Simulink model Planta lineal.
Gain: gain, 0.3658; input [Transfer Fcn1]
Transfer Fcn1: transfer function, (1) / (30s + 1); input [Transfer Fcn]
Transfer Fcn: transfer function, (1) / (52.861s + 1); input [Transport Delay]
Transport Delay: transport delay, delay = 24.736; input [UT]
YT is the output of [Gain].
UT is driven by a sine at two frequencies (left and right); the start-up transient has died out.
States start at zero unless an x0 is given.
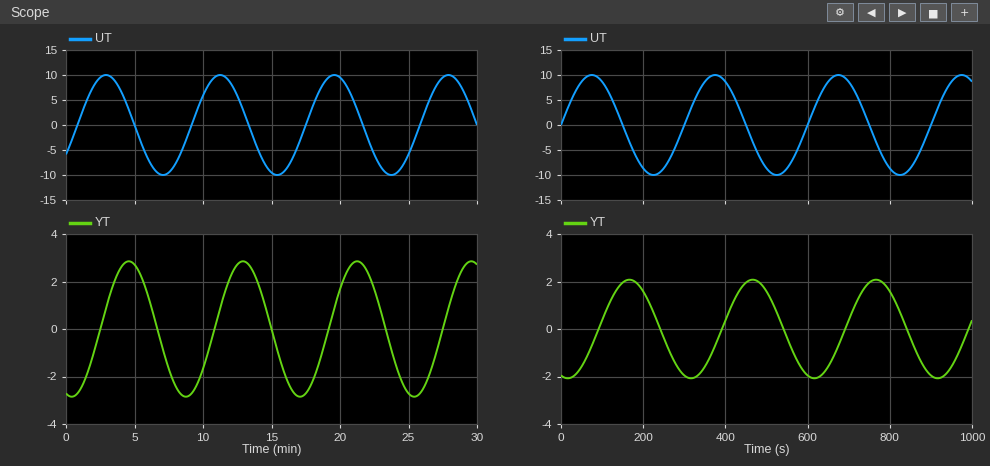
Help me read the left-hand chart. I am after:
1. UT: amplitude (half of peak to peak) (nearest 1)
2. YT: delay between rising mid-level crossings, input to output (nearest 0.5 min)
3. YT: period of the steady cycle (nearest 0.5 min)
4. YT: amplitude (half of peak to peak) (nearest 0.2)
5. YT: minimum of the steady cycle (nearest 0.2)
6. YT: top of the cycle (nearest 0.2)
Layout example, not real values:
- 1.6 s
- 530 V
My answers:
- 10
- 1.5 min
- 8.5 min
- 2.8
- -2.8
- 2.8
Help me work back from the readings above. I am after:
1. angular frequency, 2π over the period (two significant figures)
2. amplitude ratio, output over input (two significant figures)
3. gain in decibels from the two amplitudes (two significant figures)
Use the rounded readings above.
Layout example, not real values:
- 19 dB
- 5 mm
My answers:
- 0.74 rad/min
- 0.28
- -11 dB
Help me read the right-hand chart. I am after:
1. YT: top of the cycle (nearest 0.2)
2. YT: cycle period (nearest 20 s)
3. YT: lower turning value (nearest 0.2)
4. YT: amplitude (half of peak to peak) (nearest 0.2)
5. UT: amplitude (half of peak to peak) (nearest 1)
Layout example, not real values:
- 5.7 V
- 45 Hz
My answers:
- 2.0
- 300 s
- -2.0
- 2.0
- 10
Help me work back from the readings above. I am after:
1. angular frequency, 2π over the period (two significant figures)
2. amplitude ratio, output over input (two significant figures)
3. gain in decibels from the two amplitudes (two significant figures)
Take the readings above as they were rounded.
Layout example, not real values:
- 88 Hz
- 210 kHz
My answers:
- 0.021 rad/s
- 0.20
- -14 dB
